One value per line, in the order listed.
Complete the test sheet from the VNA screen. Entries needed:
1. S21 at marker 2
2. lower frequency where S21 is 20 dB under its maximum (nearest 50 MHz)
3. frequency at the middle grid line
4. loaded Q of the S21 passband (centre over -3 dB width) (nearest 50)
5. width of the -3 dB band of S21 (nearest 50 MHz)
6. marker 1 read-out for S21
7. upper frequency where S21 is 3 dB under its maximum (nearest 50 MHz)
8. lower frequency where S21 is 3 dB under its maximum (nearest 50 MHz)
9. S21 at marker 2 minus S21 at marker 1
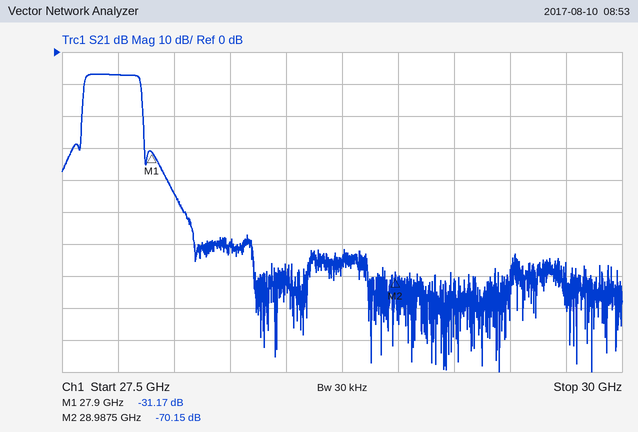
-70.15 dB
27.60 GHz
28.75 GHz
100
250 MHz
-31.17 dB
27.85 GHz
27.60 GHz
-38.98 dB
